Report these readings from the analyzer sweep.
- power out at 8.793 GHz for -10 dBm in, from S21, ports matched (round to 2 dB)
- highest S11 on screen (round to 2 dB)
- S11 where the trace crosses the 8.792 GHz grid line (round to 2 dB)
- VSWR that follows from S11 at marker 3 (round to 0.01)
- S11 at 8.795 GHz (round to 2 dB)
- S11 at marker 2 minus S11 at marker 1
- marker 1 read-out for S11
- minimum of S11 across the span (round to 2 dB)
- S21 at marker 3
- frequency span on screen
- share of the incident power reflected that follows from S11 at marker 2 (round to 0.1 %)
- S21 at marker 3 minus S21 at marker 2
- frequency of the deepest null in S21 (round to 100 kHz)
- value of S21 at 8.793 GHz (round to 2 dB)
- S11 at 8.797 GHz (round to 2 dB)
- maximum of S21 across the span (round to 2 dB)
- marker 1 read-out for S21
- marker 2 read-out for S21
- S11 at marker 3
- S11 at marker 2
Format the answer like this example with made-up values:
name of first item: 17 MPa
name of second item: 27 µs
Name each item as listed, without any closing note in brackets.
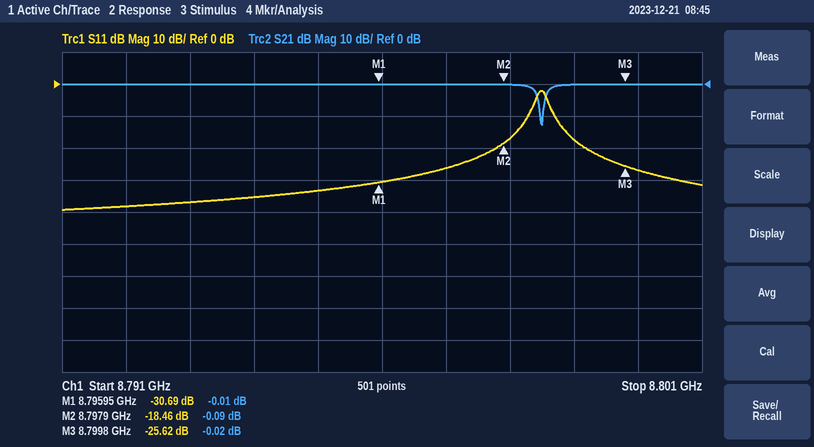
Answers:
power out at 8.793 GHz for -10 dBm in, from S21, ports matched: -10 dBm
highest S11 on screen: -2 dB
S11 where the trace crosses the 8.792 GHz grid line: -38 dB
VSWR that follows from S11 at marker 3: 1.11
S11 at 8.795 GHz: -34 dB
S11 at marker 2 minus S11 at marker 1: 12.23 dB
marker 1 read-out for S11: -30.69 dB
minimum of S11 across the span: -40 dB
S21 at marker 3: -0.02 dB
frequency span on screen: 10 MHz
share of the incident power reflected that follows from S11 at marker 2: 1.4 %
S21 at marker 3 minus S21 at marker 2: 0.07 dB
frequency of the deepest null in S21: 8.7985 GHz
value of S21 at 8.793 GHz: 0 dB
S11 at 8.797 GHz: -26 dB
maximum of S21 across the span: 0 dB
marker 1 read-out for S21: -0.01 dB
marker 2 read-out for S21: -0.09 dB
S11 at marker 3: -25.62 dB
S11 at marker 2: -18.46 dB
